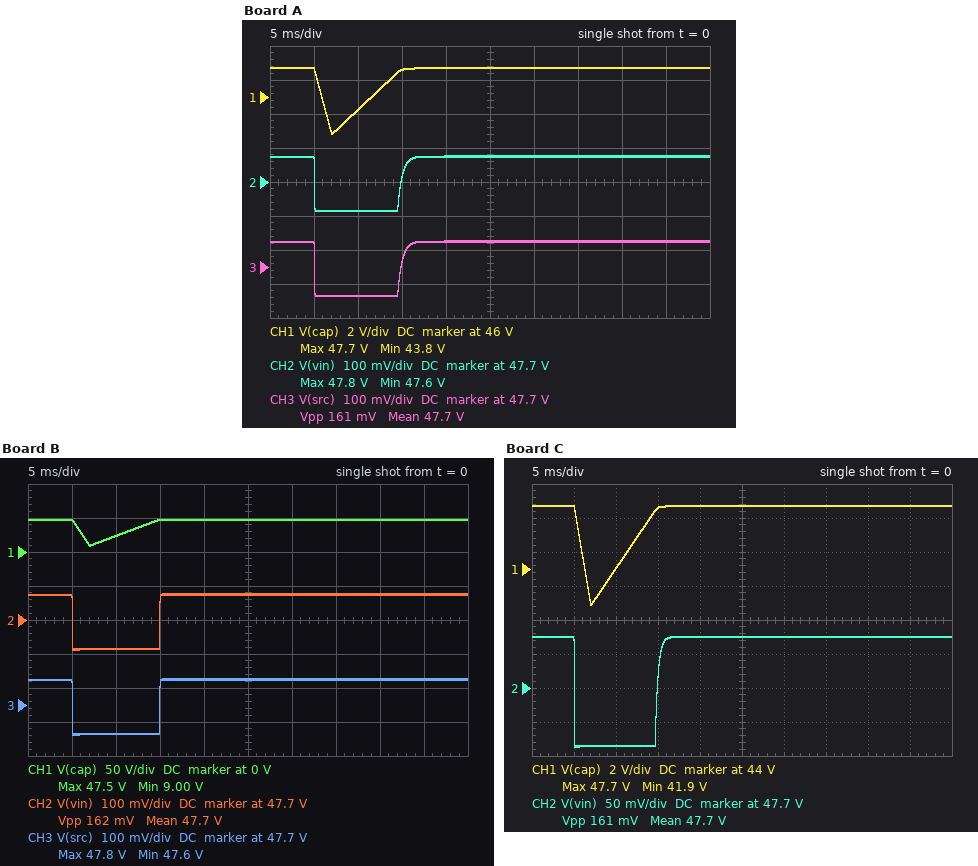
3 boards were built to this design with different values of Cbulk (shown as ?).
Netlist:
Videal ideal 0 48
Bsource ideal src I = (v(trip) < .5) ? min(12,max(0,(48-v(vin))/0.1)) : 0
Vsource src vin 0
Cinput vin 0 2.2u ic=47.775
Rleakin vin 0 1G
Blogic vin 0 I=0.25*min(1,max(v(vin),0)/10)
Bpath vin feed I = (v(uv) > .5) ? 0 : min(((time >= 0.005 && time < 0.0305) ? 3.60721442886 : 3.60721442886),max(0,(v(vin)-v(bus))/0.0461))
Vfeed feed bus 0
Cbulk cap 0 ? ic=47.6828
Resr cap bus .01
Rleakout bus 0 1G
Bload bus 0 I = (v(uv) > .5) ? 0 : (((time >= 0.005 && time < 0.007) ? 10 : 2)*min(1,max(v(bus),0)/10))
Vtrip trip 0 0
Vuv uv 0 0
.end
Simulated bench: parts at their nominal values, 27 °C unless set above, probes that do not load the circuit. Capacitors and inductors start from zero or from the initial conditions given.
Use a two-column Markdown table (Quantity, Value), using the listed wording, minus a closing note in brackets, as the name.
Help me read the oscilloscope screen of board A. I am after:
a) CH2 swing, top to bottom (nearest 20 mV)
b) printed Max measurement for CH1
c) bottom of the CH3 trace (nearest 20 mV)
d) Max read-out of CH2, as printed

| Quantity | Value |
|---|---|
| CH2 swing, top to bottom | 160 mV |
| printed Max measurement for CH1 | 47.7 V |
| bottom of the CH3 trace | 47.62 V |
| Max read-out of CH2, as printed | 47.8 V |
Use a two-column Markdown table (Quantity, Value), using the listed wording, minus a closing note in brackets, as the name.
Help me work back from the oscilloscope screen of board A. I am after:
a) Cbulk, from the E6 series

| Quantity | Value |
|---|---|
| Cbulk, from the E6 series | 3.3 mF |
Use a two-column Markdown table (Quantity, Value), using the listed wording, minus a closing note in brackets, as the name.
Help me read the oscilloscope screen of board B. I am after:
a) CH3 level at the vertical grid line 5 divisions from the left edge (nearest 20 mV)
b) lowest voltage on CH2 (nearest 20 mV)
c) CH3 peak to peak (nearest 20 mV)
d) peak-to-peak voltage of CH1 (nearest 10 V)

| Quantity | Value |
|---|---|
| CH3 level at the vertical grid line 5 divisions from the left edge | 47.78 V |
| lowest voltage on CH2 | 47.62 V |
| CH3 peak to peak | 160 mV |
| peak-to-peak voltage of CH1 | 40 V |
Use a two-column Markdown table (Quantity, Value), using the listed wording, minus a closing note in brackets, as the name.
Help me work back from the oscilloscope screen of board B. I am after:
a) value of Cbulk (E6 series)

| Quantity | Value |
|---|---|
| value of Cbulk | 330 µF |
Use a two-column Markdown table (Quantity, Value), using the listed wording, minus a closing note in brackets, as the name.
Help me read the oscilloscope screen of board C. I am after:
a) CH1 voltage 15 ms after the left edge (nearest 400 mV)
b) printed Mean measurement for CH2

| Quantity | Value |
|---|---|
| CH1 voltage 15 ms after the left edge | 47.6 V |
| printed Mean measurement for CH2 | 47.7 V |
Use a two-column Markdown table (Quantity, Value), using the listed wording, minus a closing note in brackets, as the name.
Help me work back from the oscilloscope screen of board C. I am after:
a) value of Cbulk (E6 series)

| Quantity | Value |
|---|---|
| value of Cbulk | 2.2 mF |
